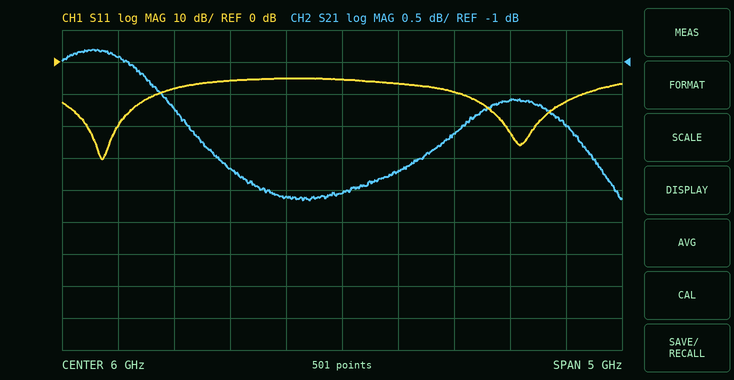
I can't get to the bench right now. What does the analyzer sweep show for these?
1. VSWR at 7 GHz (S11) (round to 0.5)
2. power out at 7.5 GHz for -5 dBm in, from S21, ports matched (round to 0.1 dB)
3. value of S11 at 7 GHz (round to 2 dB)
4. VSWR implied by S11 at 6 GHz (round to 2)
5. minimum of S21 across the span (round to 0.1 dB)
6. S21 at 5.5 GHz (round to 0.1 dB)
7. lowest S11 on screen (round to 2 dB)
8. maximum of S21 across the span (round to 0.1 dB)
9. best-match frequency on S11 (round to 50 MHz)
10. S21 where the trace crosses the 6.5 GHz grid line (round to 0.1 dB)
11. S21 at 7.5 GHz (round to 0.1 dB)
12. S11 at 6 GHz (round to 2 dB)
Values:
2.0
-6.6 dBm
-10 dB
4
-3.2 dB
-3.1 dB
-30 dB
-0.8 dB
3.85 GHz
-2.7 dB
-1.6 dB
-6 dB
